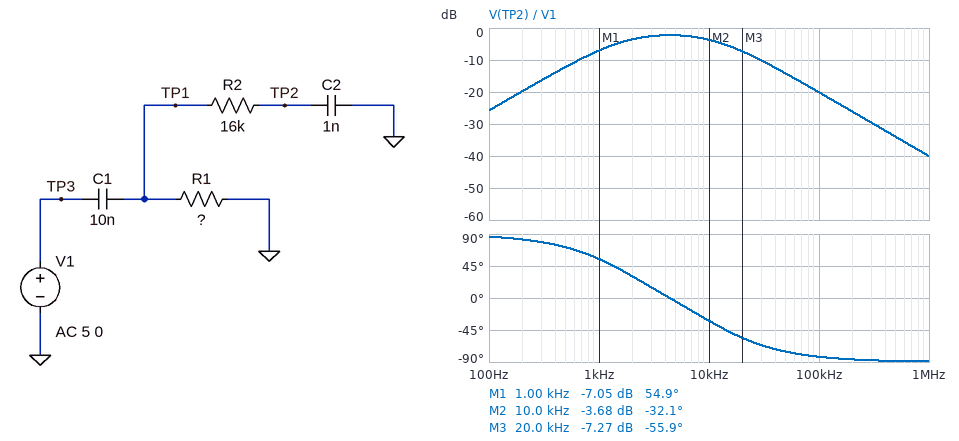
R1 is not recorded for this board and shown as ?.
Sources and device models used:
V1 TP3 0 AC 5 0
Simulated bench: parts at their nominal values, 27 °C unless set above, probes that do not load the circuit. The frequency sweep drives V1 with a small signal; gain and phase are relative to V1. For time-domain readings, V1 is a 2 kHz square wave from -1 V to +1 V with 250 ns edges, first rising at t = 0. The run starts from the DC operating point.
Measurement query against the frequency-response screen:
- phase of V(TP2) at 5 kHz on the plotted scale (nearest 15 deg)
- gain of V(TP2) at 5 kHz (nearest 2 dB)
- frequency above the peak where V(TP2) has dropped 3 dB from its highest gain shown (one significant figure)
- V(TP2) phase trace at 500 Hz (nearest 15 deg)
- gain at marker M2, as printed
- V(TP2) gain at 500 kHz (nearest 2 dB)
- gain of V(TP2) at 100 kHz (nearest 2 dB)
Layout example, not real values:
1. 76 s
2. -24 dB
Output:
1. 0 deg
2. -2 dB
3. 10 kHz
4. 75 deg
5. -3.68 dB
6. -34 dB
7. -20 dB
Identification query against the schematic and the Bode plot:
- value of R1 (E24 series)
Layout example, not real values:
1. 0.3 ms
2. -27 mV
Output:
1. 8.2 kΩ
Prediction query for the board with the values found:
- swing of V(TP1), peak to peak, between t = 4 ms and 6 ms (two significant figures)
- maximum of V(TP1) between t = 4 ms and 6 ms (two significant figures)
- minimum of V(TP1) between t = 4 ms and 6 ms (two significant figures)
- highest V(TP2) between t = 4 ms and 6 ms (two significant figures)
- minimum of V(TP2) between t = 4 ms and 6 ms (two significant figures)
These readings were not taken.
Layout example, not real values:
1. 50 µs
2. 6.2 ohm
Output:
1. 3.8 V
2. 1.9 V
3. -1.9 V
4. 1.2 V
5. -1.2 V
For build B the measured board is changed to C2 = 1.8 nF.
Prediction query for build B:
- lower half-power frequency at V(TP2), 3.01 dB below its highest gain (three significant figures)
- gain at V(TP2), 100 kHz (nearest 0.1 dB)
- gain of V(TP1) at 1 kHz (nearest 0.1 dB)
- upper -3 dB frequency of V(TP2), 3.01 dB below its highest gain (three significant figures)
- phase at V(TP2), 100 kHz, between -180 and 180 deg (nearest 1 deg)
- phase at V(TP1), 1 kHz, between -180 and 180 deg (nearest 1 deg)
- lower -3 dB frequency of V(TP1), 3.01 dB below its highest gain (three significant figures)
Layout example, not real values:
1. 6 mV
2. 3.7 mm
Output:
1. 1.12 kHz
2. -25.2 dB
3. -7.2 dB
4. 9.58 kHz
5. -85 deg
6. 59 deg
7. 2.56 kHz
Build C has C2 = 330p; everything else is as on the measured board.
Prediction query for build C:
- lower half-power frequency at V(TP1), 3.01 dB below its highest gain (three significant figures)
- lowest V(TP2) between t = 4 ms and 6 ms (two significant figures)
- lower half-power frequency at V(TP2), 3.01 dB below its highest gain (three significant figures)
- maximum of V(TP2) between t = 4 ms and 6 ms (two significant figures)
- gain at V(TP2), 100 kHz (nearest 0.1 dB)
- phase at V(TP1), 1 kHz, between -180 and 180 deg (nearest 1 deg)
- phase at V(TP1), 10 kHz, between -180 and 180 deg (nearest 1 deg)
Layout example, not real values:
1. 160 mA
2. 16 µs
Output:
1. 2.01 kHz
2. -1.5 V
3. 1.68 kHz
4. 1.5 V
5. -10.8 dB
6. 62 deg
7. 11 deg
